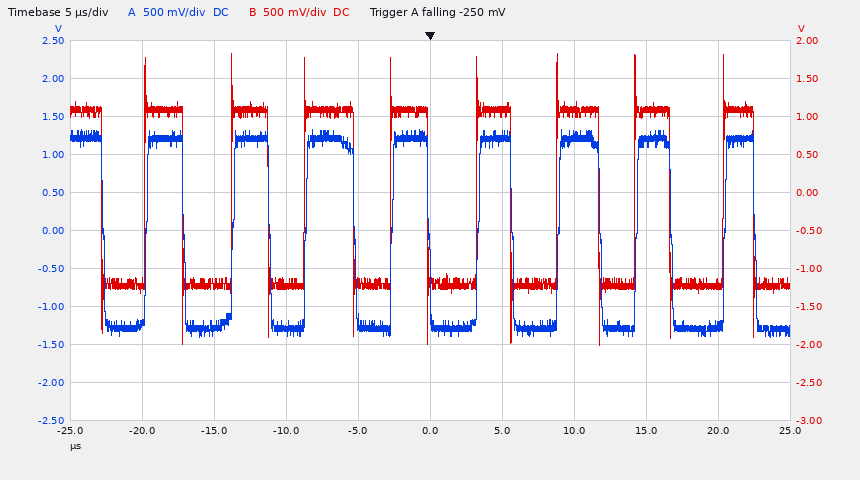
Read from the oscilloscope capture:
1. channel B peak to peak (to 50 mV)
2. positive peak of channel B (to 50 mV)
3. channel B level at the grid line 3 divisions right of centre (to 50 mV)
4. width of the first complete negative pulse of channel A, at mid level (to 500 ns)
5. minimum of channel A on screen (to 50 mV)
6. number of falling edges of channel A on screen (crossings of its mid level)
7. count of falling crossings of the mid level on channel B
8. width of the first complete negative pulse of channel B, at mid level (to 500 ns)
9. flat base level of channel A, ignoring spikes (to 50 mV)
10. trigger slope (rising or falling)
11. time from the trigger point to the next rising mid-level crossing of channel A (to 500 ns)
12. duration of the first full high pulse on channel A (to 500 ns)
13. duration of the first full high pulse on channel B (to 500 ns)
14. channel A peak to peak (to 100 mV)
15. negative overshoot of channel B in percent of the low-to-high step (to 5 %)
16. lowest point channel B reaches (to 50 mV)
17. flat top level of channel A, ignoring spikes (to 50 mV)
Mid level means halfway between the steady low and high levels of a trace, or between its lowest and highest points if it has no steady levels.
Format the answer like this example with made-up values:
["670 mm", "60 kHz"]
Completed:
["3.85 V", "1.85 V", "1.10 V", "3.0 µs", "-1.40 V", "9", "9", "3.0 µs", "-1.30 V", "falling", "3.5 µs", "2.5 µs", "2.5 µs", "2.70 V", "35 %", "-2.00 V", "1.20 V"]
